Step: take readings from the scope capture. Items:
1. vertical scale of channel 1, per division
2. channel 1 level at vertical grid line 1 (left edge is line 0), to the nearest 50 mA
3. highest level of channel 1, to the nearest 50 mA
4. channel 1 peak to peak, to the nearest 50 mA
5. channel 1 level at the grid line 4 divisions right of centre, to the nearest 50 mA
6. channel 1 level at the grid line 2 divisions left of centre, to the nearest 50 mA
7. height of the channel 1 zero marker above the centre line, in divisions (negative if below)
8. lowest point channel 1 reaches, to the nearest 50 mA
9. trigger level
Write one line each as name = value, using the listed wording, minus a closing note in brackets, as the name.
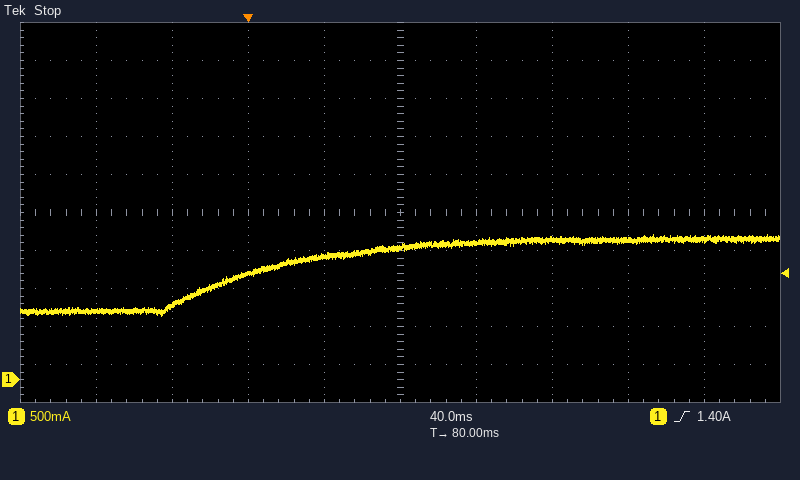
vertical scale of channel 1, per division = 500 mA
channel 1 level at vertical grid line 1 (left edge is line 0), to the nearest 50 mA = 900 mA
highest level of channel 1, to the nearest 50 mA = 1.90 A
channel 1 peak to peak, to the nearest 50 mA = 1.05 A
channel 1 level at the grid line 4 divisions right of centre, to the nearest 50 mA = 1.85 A
channel 1 level at the grid line 2 divisions left of centre, to the nearest 50 mA = 1.40 A
height of the channel 1 zero marker above the centre line, in divisions = -4.4 div
lowest point channel 1 reaches, to the nearest 50 mA = 850 mA
trigger level = 1.40 A
